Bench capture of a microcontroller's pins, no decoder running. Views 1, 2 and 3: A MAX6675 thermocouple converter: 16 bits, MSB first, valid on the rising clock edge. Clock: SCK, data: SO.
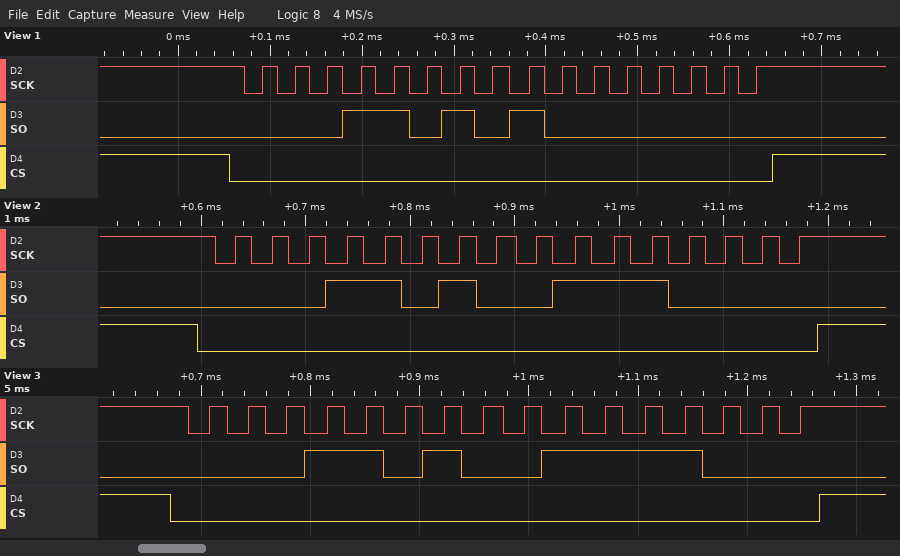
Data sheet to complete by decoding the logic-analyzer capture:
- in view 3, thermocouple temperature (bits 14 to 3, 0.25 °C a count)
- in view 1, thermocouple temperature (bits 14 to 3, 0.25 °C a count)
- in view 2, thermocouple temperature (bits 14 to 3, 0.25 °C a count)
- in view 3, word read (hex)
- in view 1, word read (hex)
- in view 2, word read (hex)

211.75 °C
212.00 °C
211.50 °C
0x1A78
0x1A80
0x1A70
